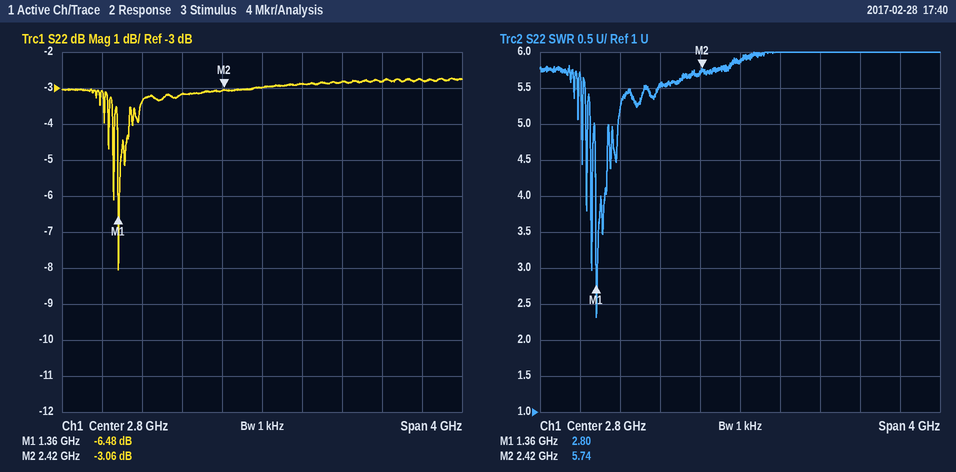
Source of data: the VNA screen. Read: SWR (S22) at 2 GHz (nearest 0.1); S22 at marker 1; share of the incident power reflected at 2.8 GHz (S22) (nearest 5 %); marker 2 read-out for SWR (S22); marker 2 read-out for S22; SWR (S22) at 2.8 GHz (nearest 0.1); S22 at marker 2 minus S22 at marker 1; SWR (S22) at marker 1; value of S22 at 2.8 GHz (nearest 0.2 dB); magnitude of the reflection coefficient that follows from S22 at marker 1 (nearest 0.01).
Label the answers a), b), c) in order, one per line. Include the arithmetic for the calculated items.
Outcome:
a) 5.5
b) -6.48 dB
c) 10^(-3/10) ≈ 50 %
d) 5.74
e) -3.06 dB
f) 5.9
g) -3.06 − (-6.48) = 3.42 dB
h) 2.80
i) -3.0 dB
j) 10^(-6.48/20) ≈ 0.47
